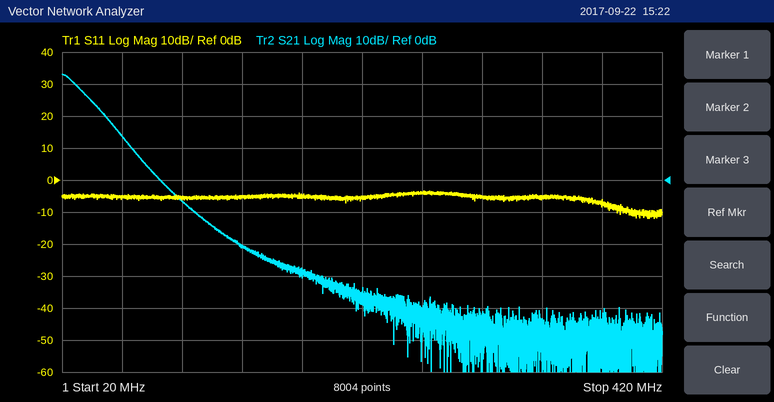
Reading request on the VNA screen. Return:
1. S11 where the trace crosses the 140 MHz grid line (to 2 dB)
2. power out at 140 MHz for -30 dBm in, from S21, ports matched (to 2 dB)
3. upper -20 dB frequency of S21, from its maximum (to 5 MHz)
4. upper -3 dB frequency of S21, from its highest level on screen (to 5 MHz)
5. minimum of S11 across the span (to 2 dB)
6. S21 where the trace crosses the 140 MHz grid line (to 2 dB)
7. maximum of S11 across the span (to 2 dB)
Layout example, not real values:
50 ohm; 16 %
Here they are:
-6 dB; -50 dBm; 60 MHz; 30 MHz; -12 dB; -20 dB; -4 dB
